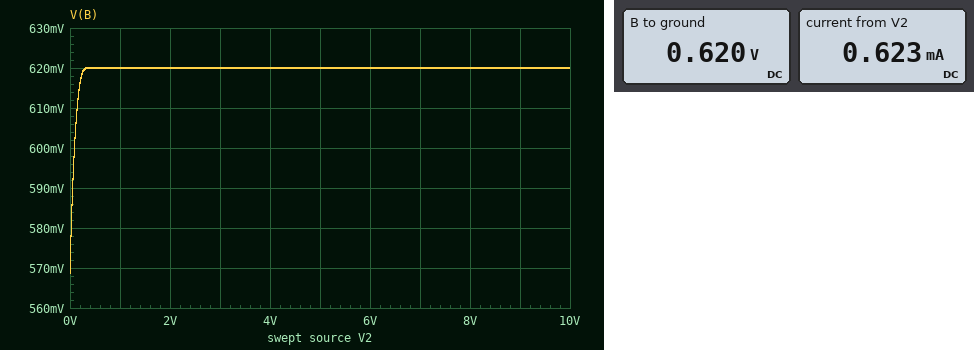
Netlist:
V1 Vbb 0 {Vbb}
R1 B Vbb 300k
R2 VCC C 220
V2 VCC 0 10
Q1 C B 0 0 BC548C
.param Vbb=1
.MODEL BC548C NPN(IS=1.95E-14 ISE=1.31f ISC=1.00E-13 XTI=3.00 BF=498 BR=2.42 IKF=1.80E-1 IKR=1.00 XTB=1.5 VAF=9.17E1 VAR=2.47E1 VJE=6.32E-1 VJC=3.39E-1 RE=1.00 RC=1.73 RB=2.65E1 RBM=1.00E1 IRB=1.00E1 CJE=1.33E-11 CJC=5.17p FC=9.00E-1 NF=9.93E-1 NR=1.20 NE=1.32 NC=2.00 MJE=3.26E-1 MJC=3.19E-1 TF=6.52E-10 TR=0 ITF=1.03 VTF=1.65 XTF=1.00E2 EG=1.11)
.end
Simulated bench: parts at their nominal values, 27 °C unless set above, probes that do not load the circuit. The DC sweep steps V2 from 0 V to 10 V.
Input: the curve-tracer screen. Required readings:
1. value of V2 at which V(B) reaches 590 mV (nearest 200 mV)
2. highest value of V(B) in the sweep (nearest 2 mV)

0 V
620 mV
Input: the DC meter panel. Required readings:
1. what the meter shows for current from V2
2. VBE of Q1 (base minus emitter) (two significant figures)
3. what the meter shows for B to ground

0.623 mA
620 mV
0.620 V
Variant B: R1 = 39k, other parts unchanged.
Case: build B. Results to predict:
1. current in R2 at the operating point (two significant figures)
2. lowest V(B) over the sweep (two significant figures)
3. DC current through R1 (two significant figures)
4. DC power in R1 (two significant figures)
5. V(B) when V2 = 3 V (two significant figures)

4.1 mA
600 mV
8.4 µA
2.7 µW
670 mV
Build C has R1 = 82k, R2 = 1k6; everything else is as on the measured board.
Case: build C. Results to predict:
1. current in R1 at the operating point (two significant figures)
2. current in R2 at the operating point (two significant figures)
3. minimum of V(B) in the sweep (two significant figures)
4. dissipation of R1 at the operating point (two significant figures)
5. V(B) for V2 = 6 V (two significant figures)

4.2 µA
2.0 mA
560 mV
1.5 µW
650 mV
